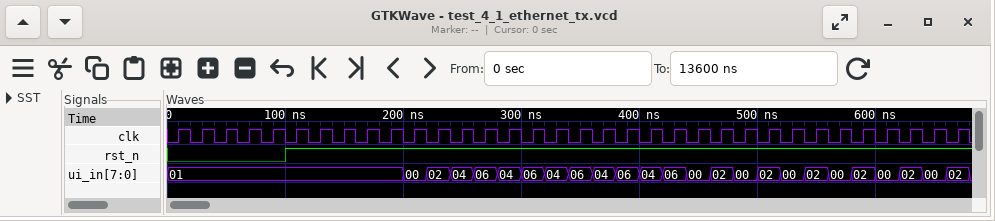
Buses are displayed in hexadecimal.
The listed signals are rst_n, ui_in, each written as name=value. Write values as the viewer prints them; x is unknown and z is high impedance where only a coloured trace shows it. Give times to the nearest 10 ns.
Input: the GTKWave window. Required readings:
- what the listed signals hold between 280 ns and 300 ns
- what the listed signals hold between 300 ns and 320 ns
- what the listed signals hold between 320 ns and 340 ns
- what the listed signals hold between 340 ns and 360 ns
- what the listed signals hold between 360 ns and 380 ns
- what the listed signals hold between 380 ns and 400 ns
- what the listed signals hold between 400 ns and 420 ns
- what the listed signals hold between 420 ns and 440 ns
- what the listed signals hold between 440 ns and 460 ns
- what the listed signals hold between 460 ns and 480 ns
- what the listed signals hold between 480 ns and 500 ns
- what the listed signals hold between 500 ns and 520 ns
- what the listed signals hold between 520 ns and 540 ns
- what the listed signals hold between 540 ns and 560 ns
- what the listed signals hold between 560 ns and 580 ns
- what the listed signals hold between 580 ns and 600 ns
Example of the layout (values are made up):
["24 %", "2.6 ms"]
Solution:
["rst_n=1, ui_in=04", "rst_n=1, ui_in=06", "rst_n=1, ui_in=04", "rst_n=1, ui_in=06", "rst_n=1, ui_in=04", "rst_n=1, ui_in=06", "rst_n=1, ui_in=04", "rst_n=1, ui_in=06", "rst_n=1, ui_in=00", "rst_n=1, ui_in=02", "rst_n=1, ui_in=00", "rst_n=1, ui_in=02", "rst_n=1, ui_in=00", "rst_n=1, ui_in=02", "rst_n=1, ui_in=00", "rst_n=1, ui_in=02"]
